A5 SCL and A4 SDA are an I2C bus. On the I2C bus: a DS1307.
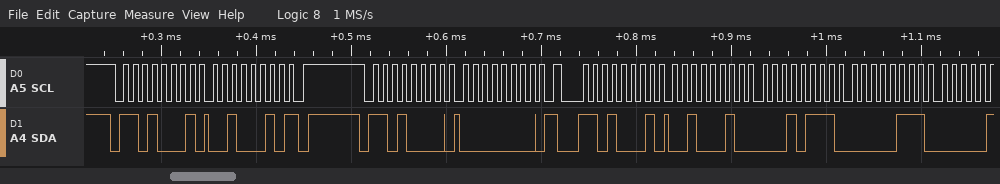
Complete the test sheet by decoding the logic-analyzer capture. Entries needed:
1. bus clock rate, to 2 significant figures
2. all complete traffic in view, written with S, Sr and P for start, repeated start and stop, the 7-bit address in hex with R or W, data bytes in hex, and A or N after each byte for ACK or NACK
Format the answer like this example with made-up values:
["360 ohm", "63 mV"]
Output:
["100 kHz", "S 68R A 22 N P S 68W A 00 A Sr 68R A 22 A 17 A 07 A"]
